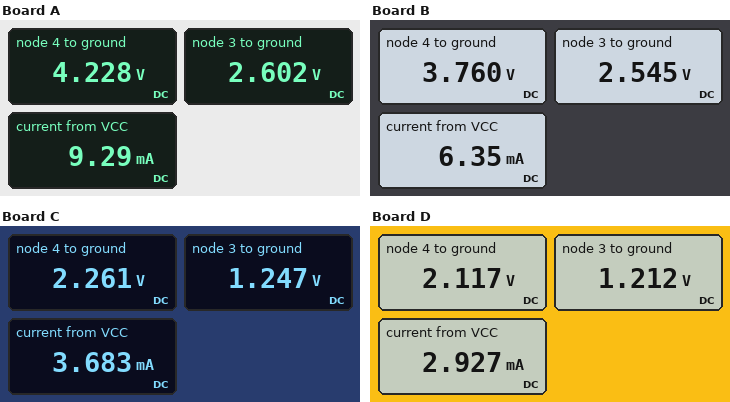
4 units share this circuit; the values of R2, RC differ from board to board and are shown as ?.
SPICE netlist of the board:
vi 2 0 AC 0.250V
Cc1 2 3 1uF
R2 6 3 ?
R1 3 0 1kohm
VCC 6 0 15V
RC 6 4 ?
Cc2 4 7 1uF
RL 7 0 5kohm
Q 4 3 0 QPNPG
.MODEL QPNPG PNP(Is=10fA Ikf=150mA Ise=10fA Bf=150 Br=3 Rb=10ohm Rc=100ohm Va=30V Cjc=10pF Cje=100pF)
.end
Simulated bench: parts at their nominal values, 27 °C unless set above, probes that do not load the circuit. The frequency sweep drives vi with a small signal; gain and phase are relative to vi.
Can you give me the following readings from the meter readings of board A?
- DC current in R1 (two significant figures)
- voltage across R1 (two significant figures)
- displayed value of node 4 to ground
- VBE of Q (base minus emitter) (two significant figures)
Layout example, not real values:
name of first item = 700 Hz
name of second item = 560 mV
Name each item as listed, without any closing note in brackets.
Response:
DC current in R1 = 2.6 mA
voltage across R1 = 2.6 V
displayed value of node 4 to ground = 4.228 V
VBE of Q (base minus emitter) = 2.6 V
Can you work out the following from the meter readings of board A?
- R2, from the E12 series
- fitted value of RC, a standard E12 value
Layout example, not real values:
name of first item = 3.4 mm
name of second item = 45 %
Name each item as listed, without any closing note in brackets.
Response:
R2, from the E12 series = 39 kΩ
fitted value of RC, a standard E12 value = 1.2 kΩ
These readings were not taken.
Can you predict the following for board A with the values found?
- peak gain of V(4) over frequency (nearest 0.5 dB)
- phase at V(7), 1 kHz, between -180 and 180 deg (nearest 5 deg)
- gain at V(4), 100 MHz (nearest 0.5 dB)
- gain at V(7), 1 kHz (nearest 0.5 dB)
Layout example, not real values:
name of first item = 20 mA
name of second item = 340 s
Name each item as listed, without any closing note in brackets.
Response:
peak gain of V(4) over frequency = -1.0 dB
phase at V(7), 1 kHz, between -180 and 180 deg = 15 deg
gain at V(4), 100 MHz = -1.5 dB
gain at V(7), 1 kHz = -1.0 dB
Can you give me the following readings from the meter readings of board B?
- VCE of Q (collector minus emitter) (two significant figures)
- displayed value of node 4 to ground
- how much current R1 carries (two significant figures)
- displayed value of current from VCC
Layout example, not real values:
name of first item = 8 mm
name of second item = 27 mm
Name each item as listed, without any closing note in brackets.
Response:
VCE of Q (collector minus emitter) = 3.8 V
displayed value of node 4 to ground = 3.760 V
how much current R1 carries = 2.5 mA
displayed value of current from VCC = 6.35 mA
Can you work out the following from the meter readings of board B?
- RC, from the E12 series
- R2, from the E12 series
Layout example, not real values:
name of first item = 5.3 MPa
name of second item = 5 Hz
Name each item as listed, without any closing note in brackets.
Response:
RC, from the E12 series = 2.2 kΩ
R2, from the E12 series = 10 kΩ
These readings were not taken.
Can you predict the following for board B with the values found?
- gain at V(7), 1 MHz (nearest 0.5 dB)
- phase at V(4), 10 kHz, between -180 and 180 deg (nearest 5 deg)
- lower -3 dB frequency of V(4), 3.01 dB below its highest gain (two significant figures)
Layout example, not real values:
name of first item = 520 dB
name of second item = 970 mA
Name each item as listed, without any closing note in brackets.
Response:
gain at V(7), 1 MHz = -0.5 dB
phase at V(4), 10 kHz, between -180 and 180 deg = 0 deg
lower -3 dB frequency of V(4), 3.01 dB below its highest gain = 200 Hz
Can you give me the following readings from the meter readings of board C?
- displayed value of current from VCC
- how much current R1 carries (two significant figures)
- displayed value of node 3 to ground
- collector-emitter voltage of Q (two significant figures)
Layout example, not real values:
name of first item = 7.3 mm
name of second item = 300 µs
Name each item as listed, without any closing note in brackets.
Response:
displayed value of current from VCC = 3.683 mA
how much current R1 carries = 1.2 mA
displayed value of node 3 to ground = 1.247 V
collector-emitter voltage of Q = 2.3 V
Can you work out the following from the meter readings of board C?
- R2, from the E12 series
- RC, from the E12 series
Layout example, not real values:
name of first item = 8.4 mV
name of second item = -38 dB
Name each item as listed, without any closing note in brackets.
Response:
R2, from the E12 series = 33 kΩ
RC, from the E12 series = 3.9 kΩ
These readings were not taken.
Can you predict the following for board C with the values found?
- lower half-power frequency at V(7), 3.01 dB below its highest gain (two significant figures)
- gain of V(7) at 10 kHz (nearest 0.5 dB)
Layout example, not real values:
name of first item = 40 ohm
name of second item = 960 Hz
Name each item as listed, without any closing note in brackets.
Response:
lower half-power frequency at V(7), 3.01 dB below its highest gain = 190 Hz
gain of V(7) at 10 kHz = -0.5 dB
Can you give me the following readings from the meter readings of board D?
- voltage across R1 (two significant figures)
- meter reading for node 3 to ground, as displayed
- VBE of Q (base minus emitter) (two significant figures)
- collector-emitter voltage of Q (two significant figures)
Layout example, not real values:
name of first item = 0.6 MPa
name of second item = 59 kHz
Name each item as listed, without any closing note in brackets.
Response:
voltage across R1 = 1.2 V
meter reading for node 3 to ground, as displayed = 1.212 V
VBE of Q (base minus emitter) = 1.2 V
collector-emitter voltage of Q = 2.1 V
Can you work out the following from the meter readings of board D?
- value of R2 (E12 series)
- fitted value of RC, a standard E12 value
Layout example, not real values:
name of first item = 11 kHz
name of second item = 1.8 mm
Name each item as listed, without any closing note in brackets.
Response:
value of R2 = 22 kΩ
fitted value of RC, a standard E12 value = 5.6 kΩ
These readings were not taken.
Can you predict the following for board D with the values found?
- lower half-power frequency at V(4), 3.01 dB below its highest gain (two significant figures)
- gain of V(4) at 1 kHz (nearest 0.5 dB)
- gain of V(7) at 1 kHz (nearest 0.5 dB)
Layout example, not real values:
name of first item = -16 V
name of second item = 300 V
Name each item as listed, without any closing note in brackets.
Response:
lower half-power frequency at V(4), 3.01 dB below its highest gain = 180 Hz
gain of V(4) at 1 kHz = -0.5 dB
gain of V(7) at 1 kHz = -0.5 dB
